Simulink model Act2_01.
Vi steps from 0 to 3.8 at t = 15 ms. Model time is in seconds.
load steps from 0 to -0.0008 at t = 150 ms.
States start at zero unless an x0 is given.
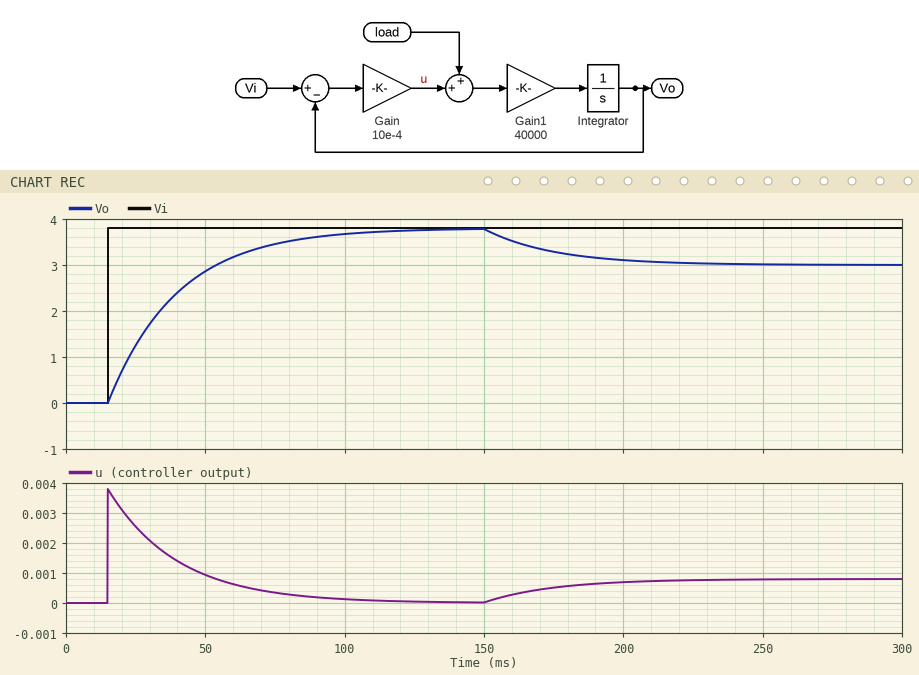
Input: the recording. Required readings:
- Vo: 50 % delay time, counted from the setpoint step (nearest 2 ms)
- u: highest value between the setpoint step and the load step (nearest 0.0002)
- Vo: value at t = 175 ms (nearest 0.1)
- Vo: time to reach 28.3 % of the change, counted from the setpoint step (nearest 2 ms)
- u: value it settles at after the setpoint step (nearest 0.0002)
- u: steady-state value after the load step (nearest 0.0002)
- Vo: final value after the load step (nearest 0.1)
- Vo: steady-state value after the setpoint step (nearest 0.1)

18 ms
0.0038
3.3
8 ms
0.0000
0.0008
3.0
3.8
